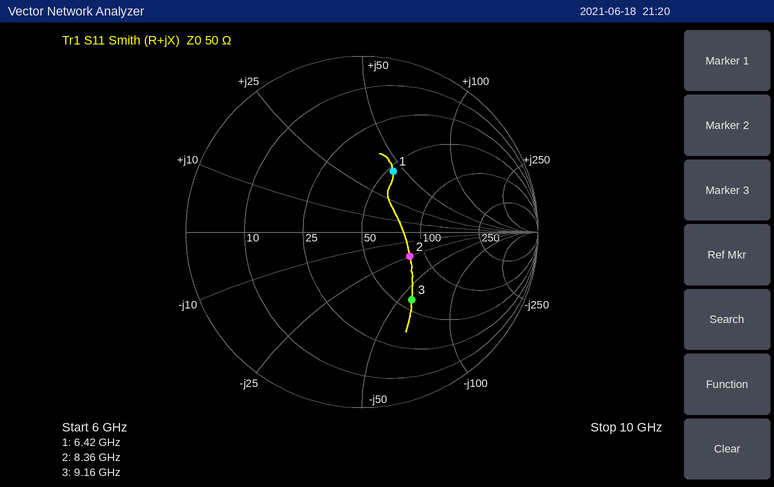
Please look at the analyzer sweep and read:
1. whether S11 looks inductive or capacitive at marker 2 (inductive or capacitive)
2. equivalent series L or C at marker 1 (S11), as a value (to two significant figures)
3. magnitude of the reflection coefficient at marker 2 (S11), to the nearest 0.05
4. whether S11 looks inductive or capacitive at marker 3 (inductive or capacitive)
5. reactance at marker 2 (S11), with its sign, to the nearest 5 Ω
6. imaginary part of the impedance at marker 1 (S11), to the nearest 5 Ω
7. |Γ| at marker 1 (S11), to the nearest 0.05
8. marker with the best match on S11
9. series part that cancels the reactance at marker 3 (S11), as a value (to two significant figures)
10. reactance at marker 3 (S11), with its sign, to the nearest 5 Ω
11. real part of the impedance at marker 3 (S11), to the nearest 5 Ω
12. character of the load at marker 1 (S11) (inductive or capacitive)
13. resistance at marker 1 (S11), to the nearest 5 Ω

capacitive
1.1 nH
0.30
capacitive
-25 Ω
+45 Ω
0.40
marker 2
1.0 nH
-60 Ω
60 Ω
inductive
55 Ω
